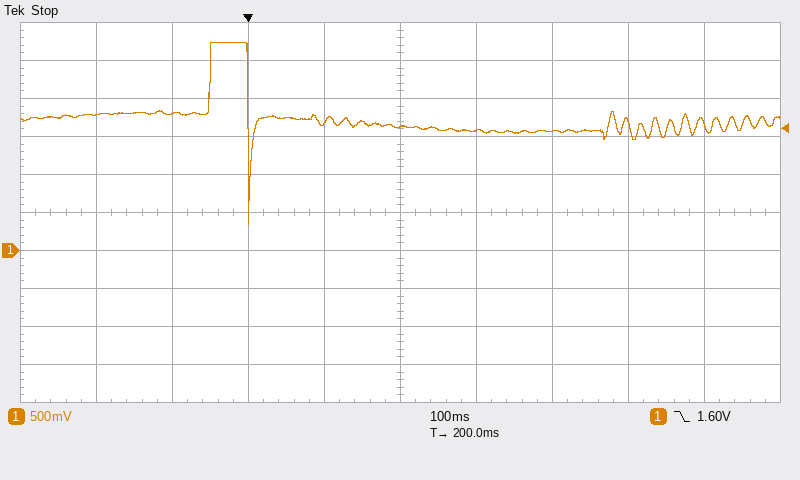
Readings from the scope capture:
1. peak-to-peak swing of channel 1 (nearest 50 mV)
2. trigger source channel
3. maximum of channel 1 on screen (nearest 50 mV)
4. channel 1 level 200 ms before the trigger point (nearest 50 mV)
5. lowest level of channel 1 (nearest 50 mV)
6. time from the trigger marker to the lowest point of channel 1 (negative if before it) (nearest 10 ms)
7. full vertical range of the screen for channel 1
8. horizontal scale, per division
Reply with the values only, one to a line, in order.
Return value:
2.40 V
channel 1
2.75 V
1.80 V
350 mV
0 ms
5 V
100 ms
